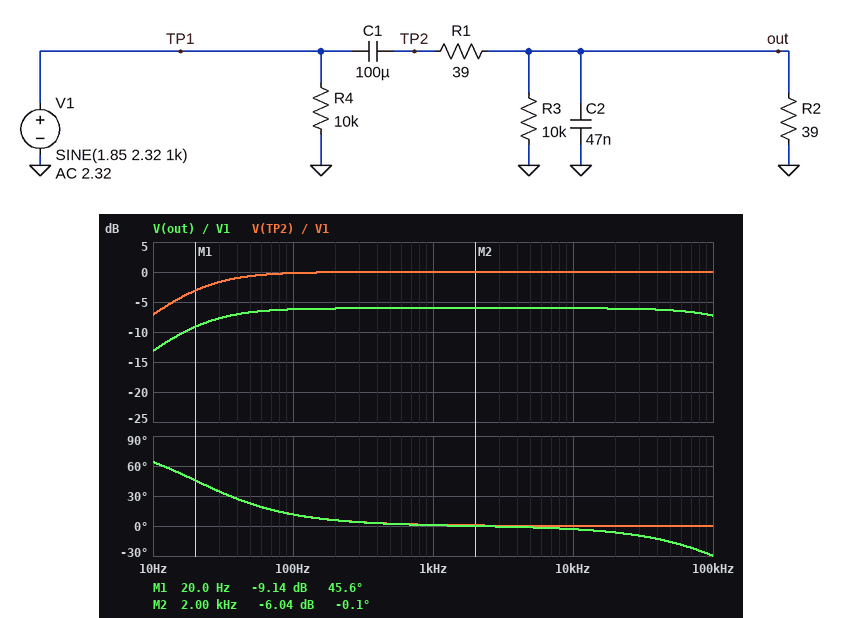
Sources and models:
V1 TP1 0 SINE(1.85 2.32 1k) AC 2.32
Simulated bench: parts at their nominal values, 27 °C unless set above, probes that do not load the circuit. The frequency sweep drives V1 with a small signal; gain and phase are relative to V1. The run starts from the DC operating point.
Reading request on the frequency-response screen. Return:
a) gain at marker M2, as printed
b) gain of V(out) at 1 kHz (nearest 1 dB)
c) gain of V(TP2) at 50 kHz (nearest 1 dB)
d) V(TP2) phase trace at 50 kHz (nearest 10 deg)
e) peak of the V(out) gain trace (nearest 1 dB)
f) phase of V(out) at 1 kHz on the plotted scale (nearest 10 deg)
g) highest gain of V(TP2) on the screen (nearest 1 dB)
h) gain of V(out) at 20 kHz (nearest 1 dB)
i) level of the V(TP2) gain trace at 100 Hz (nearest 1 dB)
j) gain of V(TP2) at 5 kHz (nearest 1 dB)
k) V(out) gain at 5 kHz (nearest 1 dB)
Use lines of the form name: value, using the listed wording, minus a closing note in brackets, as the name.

gain at marker M2, as printed: -6.04 dB
gain of V(out) at 1 kHz: -6 dB
gain of V(TP2) at 50 kHz: 0 dB
V(TP2) phase trace at 50 kHz: 0 deg
peak of the V(out) gain trace: -6 dB
phase of V(out) at 1 kHz on the plotted scale: 0 deg
highest gain of V(TP2) on the screen: 0 dB
gain of V(out) at 20 kHz: -6 dB
level of the V(TP2) gain trace at 100 Hz: 0 dB
gain of V(TP2) at 5 kHz: 0 dB
V(out) gain at 5 kHz: -6 dB
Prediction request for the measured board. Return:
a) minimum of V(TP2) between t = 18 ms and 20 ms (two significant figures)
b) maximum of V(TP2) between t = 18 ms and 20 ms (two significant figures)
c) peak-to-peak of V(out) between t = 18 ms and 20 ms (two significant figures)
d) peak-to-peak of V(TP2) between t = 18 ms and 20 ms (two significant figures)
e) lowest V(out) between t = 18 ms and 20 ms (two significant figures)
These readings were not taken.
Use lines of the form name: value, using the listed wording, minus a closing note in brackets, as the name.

minimum of V(TP2) between t = 18 ms and 20 ms: -2.3 V
maximum of V(TP2) between t = 18 ms and 20 ms: 2.3 V
peak-to-peak of V(out) between t = 18 ms and 20 ms: 2.3 V
peak-to-peak of V(TP2) between t = 18 ms and 20 ms: 4.6 V
lowest V(out) between t = 18 ms and 20 ms: -1.2 V
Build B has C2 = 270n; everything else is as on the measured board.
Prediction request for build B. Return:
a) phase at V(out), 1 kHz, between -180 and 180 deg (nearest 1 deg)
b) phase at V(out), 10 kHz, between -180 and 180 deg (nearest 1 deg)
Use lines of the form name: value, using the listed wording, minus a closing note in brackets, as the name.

phase at V(out), 1 kHz, between -180 and 180 deg: -1 deg
phase at V(out), 10 kHz, between -180 and 180 deg: -18 deg
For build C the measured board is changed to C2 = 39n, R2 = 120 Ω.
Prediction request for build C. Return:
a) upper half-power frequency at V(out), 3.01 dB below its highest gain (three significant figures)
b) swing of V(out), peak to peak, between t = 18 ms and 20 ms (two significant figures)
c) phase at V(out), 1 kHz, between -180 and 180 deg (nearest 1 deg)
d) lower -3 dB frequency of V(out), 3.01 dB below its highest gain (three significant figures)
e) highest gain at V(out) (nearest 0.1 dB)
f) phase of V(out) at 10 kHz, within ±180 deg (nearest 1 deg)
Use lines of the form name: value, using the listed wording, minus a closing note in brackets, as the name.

upper half-power frequency at V(out), 3.01 dB below its highest gain: 139 kHz
swing of V(out), peak to peak, between t = 18 ms and 20 ms: 3.5 V
phase at V(out), 1 kHz, between -180 and 180 deg: 0 deg
lower -3 dB frequency of V(out), 3.01 dB below its highest gain: 10.1 Hz
highest gain at V(out): -2.5 dB
phase of V(out) at 10 kHz, within ±180 deg: -4 deg
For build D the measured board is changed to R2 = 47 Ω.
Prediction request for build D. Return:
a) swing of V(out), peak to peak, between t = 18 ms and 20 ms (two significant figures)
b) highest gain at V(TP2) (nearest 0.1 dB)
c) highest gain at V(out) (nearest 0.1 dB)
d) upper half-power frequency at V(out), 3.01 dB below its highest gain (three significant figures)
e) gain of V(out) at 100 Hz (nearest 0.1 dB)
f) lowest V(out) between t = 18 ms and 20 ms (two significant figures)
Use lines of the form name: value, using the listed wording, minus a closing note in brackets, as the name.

swing of V(out), peak to peak, between t = 18 ms and 20 ms: 2.5 V
highest gain at V(TP2): 0 dB
highest gain at V(out): -5.3 dB
upper half-power frequency at V(out), 3.01 dB below its highest gain: 159 kHz
gain of V(out) at 100 Hz: -5.4 dB
lowest V(out) between t = 18 ms and 20 ms: -1.3 V
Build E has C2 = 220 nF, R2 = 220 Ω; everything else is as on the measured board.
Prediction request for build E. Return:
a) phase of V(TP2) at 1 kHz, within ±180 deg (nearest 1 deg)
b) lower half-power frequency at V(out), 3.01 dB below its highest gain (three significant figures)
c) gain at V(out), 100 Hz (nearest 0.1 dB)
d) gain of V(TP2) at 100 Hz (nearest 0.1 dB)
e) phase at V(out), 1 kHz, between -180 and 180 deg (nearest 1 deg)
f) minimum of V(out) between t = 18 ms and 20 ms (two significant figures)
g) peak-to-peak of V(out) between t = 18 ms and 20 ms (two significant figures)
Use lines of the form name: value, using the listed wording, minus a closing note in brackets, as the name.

phase of V(TP2) at 1 kHz, within ±180 deg: 0 deg
lower half-power frequency at V(out), 3.01 dB below its highest gain: 6.25 Hz
gain at V(out), 100 Hz: -1.5 dB
gain of V(TP2) at 100 Hz: 0 dB
phase at V(out), 1 kHz, between -180 and 180 deg: -2 deg
minimum of V(out) between t = 18 ms and 20 ms: -2.0 V
peak-to-peak of V(out) between t = 18 ms and 20 ms: 3.9 V
